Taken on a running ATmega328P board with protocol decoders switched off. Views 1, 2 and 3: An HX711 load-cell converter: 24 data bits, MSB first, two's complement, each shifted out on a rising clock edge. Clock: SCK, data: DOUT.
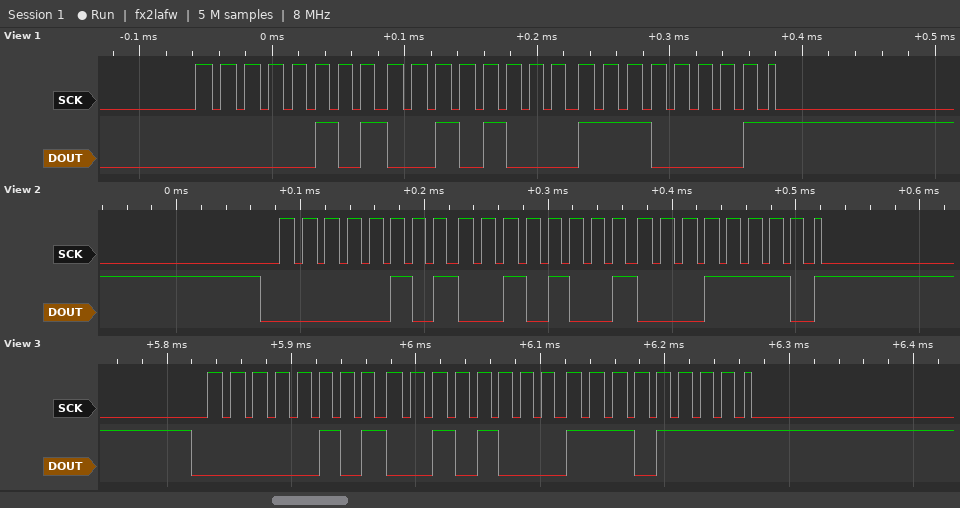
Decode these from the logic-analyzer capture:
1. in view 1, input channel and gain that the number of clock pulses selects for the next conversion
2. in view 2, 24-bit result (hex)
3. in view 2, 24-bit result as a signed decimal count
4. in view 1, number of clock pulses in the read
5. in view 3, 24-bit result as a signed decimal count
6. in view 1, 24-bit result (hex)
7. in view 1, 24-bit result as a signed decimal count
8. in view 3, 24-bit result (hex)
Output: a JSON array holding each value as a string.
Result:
["channel A, gain 128", "0x05291E", "338206", "25", "338159", "0x0528E1", "338145", "0x0528EF"]
